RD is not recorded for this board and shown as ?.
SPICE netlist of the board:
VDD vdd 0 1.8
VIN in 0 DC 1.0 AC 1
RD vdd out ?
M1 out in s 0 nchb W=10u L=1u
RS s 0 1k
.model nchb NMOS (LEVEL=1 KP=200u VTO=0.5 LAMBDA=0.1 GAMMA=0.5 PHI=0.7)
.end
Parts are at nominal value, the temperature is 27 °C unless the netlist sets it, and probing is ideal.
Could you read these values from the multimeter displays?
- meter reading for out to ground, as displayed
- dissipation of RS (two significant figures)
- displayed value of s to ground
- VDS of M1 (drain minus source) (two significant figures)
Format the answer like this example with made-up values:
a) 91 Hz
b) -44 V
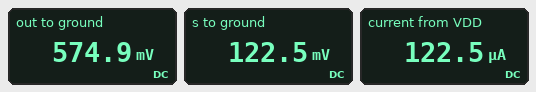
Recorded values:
a) 574.9 mV
b) 15 µW
c) 122.5 mV
d) 450 mV
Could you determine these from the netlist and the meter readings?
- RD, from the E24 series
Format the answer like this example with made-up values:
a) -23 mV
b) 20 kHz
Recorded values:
a) 10 kΩ
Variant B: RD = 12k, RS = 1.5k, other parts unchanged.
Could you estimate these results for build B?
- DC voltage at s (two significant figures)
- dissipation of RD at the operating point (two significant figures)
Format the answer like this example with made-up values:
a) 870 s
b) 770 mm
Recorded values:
a) 150 mV
b) 120 µW
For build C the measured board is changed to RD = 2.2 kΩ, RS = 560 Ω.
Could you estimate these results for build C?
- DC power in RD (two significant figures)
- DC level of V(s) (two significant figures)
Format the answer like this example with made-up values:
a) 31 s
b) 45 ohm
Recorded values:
a) 60 µW
b) 92 mV
